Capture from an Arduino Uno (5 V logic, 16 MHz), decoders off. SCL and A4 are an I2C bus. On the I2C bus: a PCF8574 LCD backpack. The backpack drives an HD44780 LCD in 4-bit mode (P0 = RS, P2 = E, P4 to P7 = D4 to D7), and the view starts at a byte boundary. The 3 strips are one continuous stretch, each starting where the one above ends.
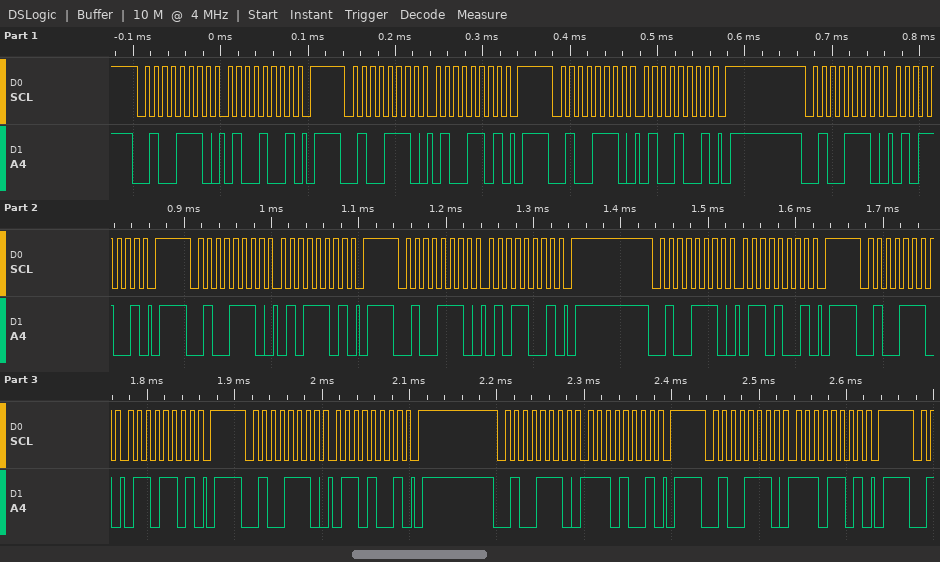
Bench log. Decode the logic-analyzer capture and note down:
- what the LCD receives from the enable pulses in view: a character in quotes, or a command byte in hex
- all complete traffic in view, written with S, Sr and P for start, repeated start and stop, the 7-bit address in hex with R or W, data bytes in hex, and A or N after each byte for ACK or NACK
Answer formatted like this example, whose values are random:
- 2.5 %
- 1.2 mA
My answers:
- 'E'
- S 27W A 49 A P S 27W A 4D A P S 27W A 49 A P S 27W A 59 A P S 27W A 5D A P S 27W A 59 A P S 27W A 69 A P S 27W A 6D A P S 27W A 69 A P S 27W A E9 A P S 27W A ED A P
